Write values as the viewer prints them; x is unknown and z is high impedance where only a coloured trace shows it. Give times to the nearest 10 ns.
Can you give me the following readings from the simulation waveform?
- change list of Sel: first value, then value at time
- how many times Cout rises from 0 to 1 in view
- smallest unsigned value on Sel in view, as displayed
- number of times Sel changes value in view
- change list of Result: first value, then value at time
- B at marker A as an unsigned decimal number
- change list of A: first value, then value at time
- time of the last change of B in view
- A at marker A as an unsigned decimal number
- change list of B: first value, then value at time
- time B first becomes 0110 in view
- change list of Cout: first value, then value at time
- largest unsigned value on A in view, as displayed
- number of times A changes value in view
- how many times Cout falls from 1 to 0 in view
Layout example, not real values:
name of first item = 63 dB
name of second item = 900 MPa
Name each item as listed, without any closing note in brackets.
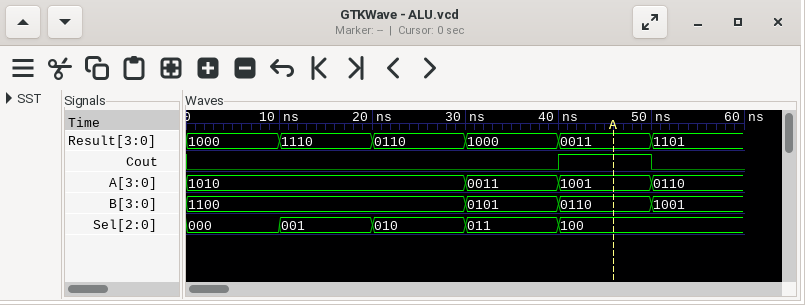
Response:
change list of Sel: first value, then value at time = 000, 001 at 10 ns, 010 at 20 ns, 011 at 30 ns, 100 at 40 ns
how many times Cout rises from 0 to 1 in view = 1
smallest unsigned value on Sel in view, as displayed = 000
number of times Sel changes value in view = 4
change list of Result: first value, then value at time = 1000, 1110 at 10 ns, 0110 at 20 ns, 1000 at 30 ns, 0011 at 40 ns, 1101 at 50 ns
B at marker A as an unsigned decimal number = 6
change list of A: first value, then value at time = 1010, 0011 at 30 ns, 1001 at 40 ns, 0110 at 50 ns
time of the last change of B in view = 50 ns
A at marker A as an unsigned decimal number = 9
change list of B: first value, then value at time = 1100, 0101 at 30 ns, 0110 at 40 ns, 1001 at 50 ns
time B first becomes 0110 in view = 40 ns
change list of Cout: first value, then value at time = 0, 1 at 40 ns, 0 at 50 ns
largest unsigned value on A in view, as displayed = 1010
number of times A changes value in view = 3
how many times Cout falls from 1 to 0 in view = 1
